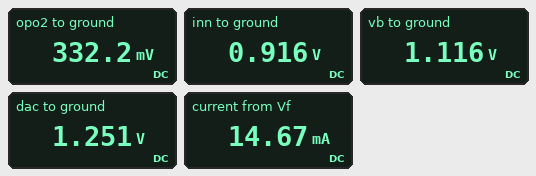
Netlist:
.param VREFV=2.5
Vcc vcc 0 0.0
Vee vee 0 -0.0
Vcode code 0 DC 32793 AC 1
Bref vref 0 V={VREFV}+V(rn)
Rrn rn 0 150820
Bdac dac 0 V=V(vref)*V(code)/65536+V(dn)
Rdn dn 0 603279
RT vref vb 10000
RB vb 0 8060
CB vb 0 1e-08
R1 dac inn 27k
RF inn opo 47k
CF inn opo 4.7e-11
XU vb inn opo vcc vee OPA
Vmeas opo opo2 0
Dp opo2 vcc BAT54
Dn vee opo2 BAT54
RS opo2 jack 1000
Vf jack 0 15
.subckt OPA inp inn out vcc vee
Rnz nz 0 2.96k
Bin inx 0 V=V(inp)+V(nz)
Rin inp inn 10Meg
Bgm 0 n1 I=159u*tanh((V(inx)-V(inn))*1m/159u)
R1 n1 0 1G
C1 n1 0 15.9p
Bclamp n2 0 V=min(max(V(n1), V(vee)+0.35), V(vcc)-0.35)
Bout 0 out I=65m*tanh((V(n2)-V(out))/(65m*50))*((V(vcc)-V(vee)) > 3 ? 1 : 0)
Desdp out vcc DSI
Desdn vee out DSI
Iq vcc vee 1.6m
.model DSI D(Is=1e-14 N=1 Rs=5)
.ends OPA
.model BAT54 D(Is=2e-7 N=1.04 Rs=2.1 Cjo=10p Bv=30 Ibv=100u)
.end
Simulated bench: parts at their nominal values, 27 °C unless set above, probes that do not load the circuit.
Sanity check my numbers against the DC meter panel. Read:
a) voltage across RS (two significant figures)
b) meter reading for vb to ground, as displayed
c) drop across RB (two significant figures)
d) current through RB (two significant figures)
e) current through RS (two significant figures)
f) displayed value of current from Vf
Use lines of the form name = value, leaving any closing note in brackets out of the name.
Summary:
voltage across RS = 15 V
meter reading for vb to ground, as displayed = 1.116 V
drop across RB = 1.1 V
current through RB = 140 µA
current through RS = 15 mA
displayed value of current from Vf = 14.67 mA
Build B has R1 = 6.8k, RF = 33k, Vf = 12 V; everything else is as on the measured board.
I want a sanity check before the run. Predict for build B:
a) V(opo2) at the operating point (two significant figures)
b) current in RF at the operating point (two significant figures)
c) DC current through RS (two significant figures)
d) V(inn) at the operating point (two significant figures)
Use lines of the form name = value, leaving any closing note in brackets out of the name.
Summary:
V(opo2) at the operating point = 320 mV
current in RF at the operating point = 23 µA
DC current through RS = 12 mA
V(inn) at the operating point = 1.1 V
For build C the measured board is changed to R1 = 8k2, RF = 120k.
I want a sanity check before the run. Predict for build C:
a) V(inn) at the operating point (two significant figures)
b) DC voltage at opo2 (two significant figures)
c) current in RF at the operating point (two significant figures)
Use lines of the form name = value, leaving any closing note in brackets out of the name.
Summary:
V(inn) at the operating point = 1.2 V
DC voltage at opo2 = 330 mV
current in RF at the operating point = 7.2 µA
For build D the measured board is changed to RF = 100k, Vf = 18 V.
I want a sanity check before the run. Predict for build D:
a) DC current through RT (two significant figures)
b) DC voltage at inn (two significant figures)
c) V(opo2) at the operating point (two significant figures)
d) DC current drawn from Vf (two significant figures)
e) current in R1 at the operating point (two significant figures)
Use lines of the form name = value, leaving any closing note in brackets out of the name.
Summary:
DC current through RT = 140 µA
DC voltage at inn = 1.1 V
V(opo2) at the operating point = 340 mV
DC current drawn from Vf = 18 mA
current in R1 at the operating point = 7.1 µA
